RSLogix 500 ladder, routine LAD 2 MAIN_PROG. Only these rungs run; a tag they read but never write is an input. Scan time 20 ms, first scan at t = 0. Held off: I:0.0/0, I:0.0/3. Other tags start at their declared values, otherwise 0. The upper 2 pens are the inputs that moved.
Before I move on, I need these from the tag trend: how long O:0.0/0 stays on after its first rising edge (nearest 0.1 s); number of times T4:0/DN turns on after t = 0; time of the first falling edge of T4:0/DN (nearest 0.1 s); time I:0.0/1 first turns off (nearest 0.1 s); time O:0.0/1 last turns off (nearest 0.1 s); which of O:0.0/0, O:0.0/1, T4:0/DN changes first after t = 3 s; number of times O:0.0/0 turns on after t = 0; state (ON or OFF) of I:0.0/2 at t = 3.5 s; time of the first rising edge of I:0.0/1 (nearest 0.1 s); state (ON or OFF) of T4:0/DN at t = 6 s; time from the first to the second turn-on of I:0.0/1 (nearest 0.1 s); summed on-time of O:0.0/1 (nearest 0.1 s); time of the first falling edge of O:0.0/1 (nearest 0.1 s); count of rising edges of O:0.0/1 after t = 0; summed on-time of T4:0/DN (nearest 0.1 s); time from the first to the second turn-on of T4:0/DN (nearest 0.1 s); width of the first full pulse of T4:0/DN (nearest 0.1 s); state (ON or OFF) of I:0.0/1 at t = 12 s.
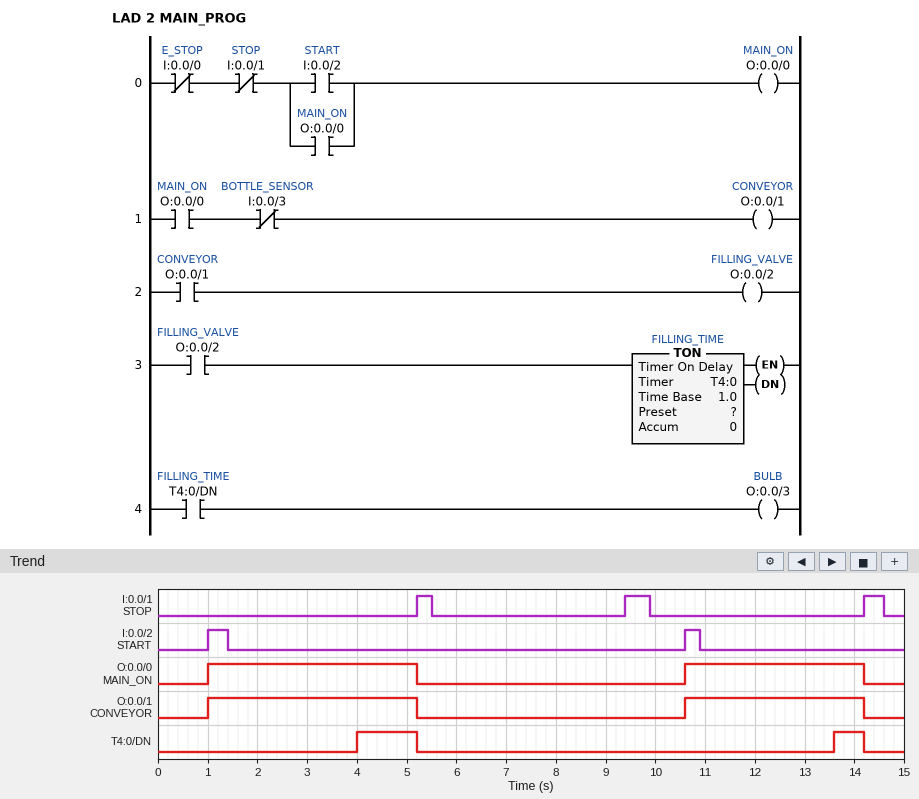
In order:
4.2 s
2
5.2 s
5.5 s
14.2 s
T4:0/DN
2
OFF
5.2 s
OFF
4.2 s
7.8 s
5.2 s
2
1.8 s
9.6 s
1.2 s
OFF
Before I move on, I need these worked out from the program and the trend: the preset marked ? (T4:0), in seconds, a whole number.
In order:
3 s
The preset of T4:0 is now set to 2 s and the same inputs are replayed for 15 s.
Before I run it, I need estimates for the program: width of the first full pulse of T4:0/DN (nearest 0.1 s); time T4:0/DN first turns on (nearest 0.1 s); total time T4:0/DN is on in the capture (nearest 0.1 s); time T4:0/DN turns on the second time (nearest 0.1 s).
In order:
2.2 s
3.0 s
3.8 s
12.6 s
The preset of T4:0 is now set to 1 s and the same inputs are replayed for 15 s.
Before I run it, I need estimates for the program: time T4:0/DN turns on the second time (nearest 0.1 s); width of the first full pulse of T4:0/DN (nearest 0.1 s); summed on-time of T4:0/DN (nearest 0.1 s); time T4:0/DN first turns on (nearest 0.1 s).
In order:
11.6 s
3.2 s
5.8 s
2.0 s
